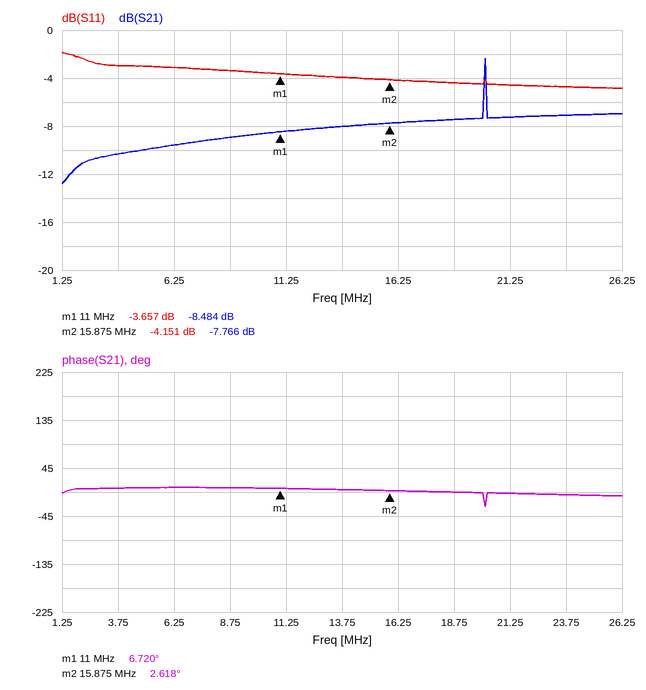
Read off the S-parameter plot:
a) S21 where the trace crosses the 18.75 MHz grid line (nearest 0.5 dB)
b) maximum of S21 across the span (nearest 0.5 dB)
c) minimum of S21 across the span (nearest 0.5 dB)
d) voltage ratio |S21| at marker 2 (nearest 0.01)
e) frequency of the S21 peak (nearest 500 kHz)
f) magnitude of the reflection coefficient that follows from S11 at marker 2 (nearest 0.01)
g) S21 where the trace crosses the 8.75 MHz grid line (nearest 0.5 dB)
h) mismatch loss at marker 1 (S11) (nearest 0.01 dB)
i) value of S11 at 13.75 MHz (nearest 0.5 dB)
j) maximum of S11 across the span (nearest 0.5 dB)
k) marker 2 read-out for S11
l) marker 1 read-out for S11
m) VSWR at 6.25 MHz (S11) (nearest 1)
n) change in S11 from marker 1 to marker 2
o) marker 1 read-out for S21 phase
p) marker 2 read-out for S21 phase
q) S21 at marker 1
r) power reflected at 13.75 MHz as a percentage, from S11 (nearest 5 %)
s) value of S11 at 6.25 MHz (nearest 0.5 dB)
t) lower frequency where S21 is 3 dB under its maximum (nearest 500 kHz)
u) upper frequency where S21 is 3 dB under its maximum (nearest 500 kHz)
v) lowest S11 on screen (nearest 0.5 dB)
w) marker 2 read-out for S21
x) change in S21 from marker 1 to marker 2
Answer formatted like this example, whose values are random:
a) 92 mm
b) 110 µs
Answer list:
a) -7.5 dB
b) -2.5 dB
c) -13.0 dB
d) 0.41
e) 20.0 MHz
f) 0.62
g) -9.0 dB
h) 2.45 dB
i) -4.0 dB
j) -2.0 dB
k) -4.151 dB
l) -3.657 dB
m) 6
n) -0.494 dB
o) 6.720°
p) 2.618°
q) -8.484 dB
r) 40 %
s) -3.0 dB
t) 20.0 MHz
u) 20.0 MHz
v) -5.0 dB
w) -7.766 dB
x) 0.718 dB
